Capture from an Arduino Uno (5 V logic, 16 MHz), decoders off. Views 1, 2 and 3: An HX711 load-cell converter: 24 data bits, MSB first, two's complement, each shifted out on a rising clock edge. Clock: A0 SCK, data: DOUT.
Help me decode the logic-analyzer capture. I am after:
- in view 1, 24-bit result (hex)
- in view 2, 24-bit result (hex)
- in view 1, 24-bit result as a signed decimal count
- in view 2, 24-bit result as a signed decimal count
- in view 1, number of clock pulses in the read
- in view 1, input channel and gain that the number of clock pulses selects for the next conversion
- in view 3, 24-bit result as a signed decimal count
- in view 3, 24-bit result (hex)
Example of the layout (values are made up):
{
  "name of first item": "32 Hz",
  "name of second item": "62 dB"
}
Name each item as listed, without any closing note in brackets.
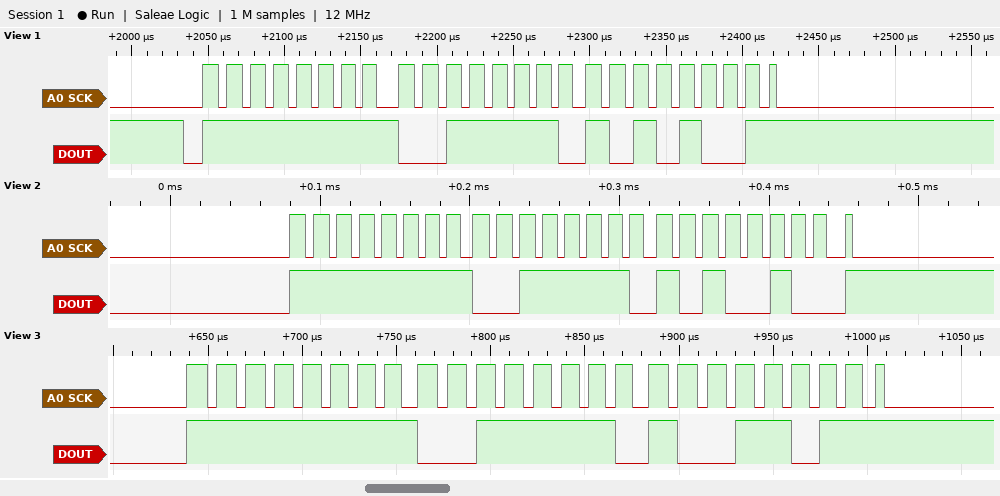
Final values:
{
  "in view 1, 24-bit result": "0xFF3EA9",
  "in view 2, 24-bit result": "0xFF3EA4",
  "in view 1, 24-bit result as a signed decimal count": "-49495",
  "in view 2, 24-bit result as a signed decimal count": "-49500",
  "in view 1, number of clock pulses in the read": "25",
  "in view 1, input channel and gain that the number of clock pulses selects for the next conversion": "channel A, gain 128",
  "in view 3, 24-bit result as a signed decimal count": "-49509",
  "in view 3, 24-bit result": "0xFF3E9B"
}
